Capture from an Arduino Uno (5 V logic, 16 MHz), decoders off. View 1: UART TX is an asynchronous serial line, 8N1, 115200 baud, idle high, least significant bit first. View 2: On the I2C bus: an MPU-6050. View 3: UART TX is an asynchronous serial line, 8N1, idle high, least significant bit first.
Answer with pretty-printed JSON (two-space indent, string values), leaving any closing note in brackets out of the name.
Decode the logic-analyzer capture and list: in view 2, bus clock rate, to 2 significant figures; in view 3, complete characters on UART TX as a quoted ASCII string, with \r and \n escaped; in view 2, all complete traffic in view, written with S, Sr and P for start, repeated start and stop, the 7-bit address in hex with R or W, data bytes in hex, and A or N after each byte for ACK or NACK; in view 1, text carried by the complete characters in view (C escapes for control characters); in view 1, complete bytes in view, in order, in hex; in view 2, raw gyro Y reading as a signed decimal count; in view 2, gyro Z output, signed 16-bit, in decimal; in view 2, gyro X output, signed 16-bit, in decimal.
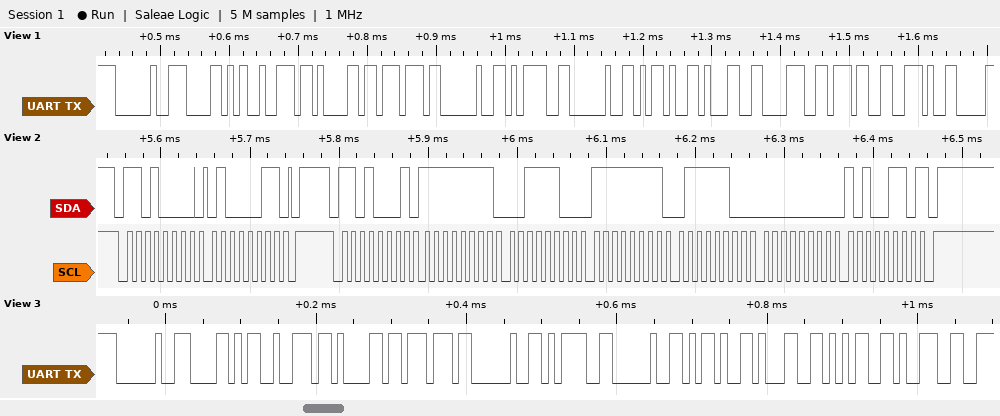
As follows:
{
  "in view 2, bus clock rate, to 2 significant figures": "100 kHz",
  "in view 3, complete characters on UART TX as a quoted ASCII string, with \\r and \\n escaped": "\" Xraw = -159\"",
  "in view 2, all complete traffic in view, written with S, Sr and P for start, repeated start and stop, the 7-bit address in hex with R or W, data bytes in hex, and A or N after each byte for ACK or NACK": "S 68W A 43 A P S 68R A FF A 3C A FF A 7C A 00 A A6 N P",
  "in view 1, text carried by the complete characters in view": "\" Xraw = -187.\"",
  "in view 1, complete bytes in view, in order, in hex": "20 58 72 61 77 20 3D 20 2D 31 38 37 2E",
  "in view 2, raw gyro Y reading as a signed decimal count": "-132",
  "in view 2, gyro Z output, signed 16-bit, in decimal": "166",
  "in view 2, gyro X output, signed 16-bit, in decimal": "-196"
}
